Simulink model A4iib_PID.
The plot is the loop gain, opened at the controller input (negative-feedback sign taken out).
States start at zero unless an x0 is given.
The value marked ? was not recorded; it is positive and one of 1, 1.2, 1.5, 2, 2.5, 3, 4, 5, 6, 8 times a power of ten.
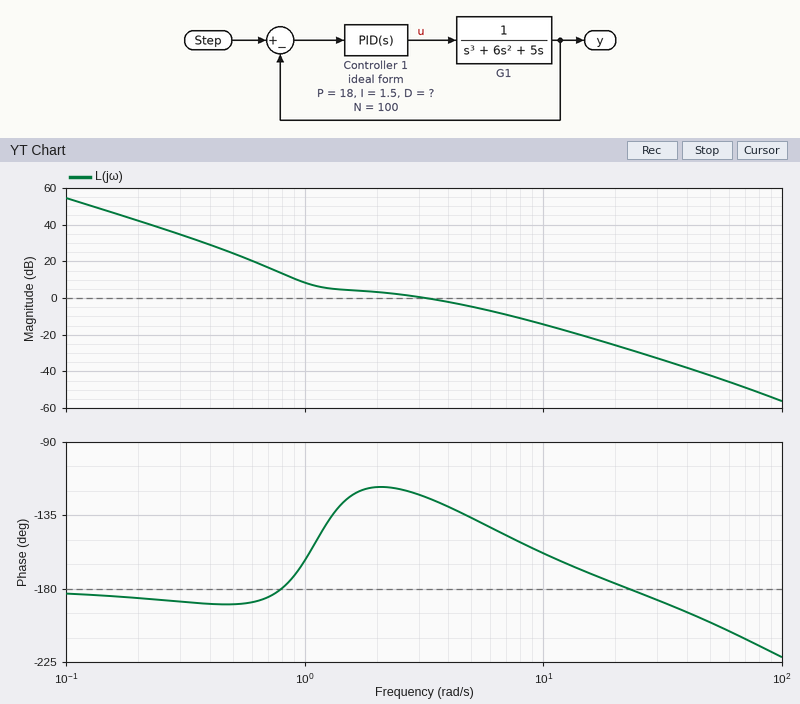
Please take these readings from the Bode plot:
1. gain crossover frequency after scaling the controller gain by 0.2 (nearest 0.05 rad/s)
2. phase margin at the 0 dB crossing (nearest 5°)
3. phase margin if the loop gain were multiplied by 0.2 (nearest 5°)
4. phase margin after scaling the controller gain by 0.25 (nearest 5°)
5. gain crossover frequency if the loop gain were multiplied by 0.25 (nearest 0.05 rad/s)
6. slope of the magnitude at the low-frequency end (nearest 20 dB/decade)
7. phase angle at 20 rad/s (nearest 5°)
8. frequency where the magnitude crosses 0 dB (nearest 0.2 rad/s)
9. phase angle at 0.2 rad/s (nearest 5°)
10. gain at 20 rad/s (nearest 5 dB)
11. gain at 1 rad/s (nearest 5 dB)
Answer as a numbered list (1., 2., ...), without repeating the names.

1. 0.80 rad/s
2. 55°
3. 0°
4. 5°
5. 0.85 rad/s
6. -40 dB/decade
7. -175°
8. 3.2 rad/s
9. -185°
10. -25 dB
11. 10 dB
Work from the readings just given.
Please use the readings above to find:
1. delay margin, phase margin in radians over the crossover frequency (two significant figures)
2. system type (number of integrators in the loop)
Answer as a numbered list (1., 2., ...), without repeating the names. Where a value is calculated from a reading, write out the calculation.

1. 55 × π / 180 / 3.2 = 0.30 s
2. 2
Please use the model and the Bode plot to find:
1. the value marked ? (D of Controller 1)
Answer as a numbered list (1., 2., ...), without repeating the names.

1. 1.2
